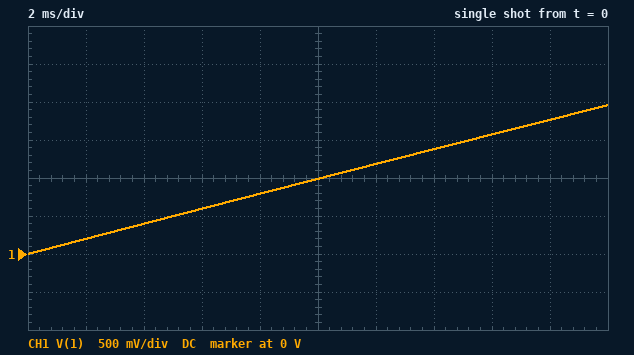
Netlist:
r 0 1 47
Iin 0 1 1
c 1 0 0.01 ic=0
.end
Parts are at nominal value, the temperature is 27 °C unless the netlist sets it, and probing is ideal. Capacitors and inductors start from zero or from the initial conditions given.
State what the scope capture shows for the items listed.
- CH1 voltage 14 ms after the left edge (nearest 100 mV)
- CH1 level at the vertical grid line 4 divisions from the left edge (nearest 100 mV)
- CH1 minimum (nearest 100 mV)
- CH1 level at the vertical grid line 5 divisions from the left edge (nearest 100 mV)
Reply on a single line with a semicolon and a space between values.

1.4 V; 800 mV; 0 V; 1.0 V
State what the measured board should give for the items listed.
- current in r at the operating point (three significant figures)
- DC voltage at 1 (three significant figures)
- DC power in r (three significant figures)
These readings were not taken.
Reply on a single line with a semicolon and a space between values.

1.00 A; 47.0 V; 47.0 W
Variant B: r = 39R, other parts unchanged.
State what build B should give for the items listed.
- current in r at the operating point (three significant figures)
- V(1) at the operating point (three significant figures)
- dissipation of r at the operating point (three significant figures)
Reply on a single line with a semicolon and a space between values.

1.00 A; 39.0 V; 39.0 W
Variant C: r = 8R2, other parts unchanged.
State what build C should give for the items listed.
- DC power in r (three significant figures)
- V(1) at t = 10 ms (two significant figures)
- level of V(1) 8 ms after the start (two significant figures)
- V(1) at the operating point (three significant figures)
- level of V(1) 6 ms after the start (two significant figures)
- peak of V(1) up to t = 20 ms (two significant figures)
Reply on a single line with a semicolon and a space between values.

8.20 W; 940 mV; 760 mV; 8.20 V; 580 mV; 1.8 V
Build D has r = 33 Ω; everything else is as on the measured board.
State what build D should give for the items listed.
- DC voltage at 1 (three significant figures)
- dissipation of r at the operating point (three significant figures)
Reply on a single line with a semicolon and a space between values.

33.0 V; 33.0 W
